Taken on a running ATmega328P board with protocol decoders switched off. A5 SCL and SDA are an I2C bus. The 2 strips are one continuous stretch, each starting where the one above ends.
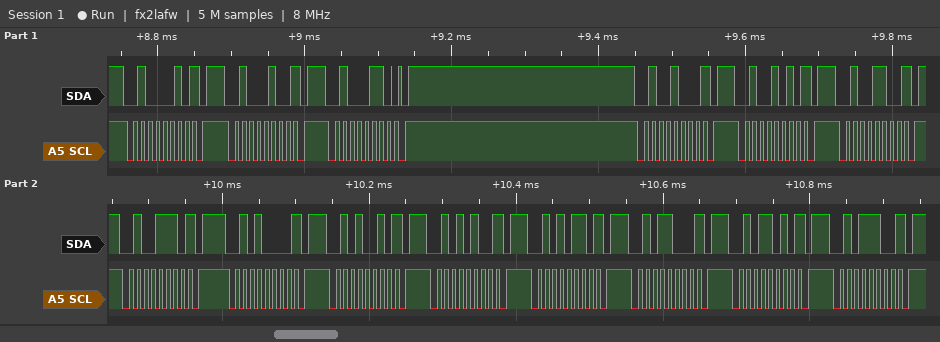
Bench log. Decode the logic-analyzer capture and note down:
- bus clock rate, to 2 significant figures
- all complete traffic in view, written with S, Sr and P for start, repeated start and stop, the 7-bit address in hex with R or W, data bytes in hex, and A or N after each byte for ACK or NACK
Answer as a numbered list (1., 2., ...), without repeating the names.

1. 100 kHz
2. S 21W N P S 22W N P S 23W A P S 24W N P S 25W N P S 26W N P S 27W N P S 28W N P S 29W N P S 2AW N P S 2BW N P S 2CW N P S 2DW N P S 2EW N P
